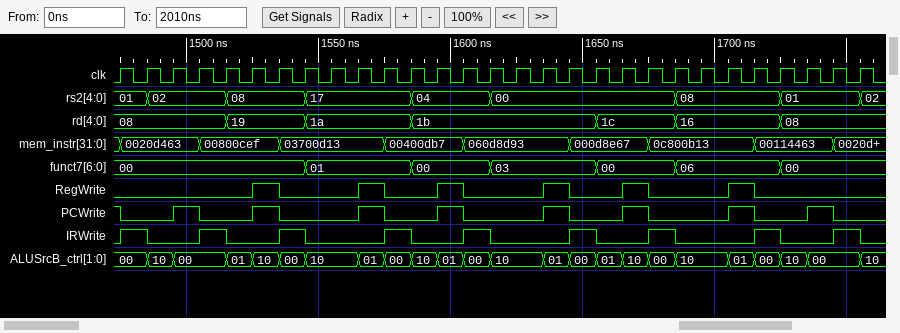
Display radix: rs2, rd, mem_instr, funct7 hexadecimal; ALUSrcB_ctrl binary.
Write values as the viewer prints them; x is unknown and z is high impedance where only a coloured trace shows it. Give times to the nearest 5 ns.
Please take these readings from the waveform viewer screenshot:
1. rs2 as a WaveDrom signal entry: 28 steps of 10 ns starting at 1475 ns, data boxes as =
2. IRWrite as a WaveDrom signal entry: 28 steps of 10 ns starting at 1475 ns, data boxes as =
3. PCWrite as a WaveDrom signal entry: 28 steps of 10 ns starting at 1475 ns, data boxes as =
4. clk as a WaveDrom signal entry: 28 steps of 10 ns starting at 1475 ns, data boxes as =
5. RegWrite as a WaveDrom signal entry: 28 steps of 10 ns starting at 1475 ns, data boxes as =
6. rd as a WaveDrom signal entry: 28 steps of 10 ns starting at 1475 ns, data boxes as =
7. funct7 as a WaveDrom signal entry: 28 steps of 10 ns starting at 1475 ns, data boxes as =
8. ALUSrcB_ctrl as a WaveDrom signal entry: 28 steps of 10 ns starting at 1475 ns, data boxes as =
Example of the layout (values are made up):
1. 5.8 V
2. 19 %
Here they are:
1. {name: 'rs2', wave: '==..=..=...=..=......=...=..', data: '01 02 08 17 04 00 08 01'}
2. {name: 'IRWrite', wave: '10.10.10..10.10..10.10..10.1'}
3. {name: 'PCWrite', wave: '0.10.10..10.10..10.10..10.10'}
4. {name: 'clk', wave: 'p...........................'}
5. {name: 'RegWrite', wave: '0....10..10.10..10.10..10...'}
6. {name: 'rd', wave: '=...=..=...=......=..=...=..', data: '08 19 1a 1b 1c 16 08'}
7. {name: 'funct7', wave: '=......=...=..=...=..=...=..', data: '00 01 00 03 00 06 00'}
8. {name: 'ALUSrcB_ctrl', wave: '===.====.======.======.====.', data: '00 10 00 01 10 00 10 01 00 10 01 00 10 01 00 01 10 00 10 01 00 10 00'}
